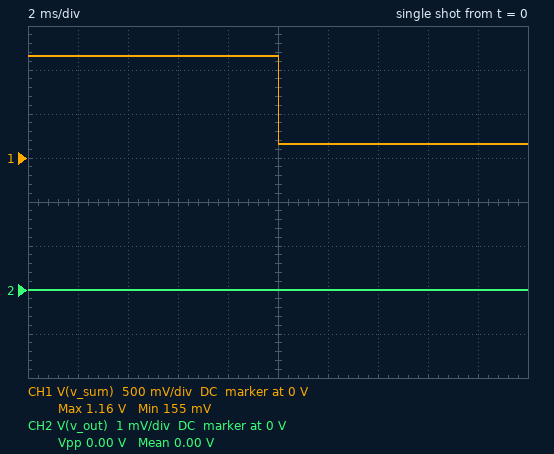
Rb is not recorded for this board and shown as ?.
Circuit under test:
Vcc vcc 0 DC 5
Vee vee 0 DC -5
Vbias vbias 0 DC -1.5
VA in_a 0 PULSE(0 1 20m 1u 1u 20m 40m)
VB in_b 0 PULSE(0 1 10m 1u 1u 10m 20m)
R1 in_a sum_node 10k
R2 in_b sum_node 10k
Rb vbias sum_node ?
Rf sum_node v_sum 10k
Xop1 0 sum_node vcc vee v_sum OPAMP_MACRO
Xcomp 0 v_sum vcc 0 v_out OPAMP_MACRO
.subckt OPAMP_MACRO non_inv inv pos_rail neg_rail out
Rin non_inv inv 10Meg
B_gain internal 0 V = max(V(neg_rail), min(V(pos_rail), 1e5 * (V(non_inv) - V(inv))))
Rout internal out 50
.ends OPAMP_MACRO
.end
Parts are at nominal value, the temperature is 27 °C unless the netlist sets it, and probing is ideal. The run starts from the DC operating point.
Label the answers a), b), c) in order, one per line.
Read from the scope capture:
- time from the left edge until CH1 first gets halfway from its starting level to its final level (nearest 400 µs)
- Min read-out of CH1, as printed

a) 10.0 ms
b) 155 mV
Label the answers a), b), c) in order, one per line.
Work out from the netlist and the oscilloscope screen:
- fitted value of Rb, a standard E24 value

a) 13 kΩ
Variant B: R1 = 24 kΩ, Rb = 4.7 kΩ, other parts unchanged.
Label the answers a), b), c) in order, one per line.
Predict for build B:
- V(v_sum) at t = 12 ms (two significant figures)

a) 2.2 V
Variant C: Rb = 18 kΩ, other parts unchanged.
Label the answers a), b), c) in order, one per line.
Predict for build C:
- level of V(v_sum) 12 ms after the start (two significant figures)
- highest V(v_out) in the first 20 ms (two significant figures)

a) -170 mV
b) 5.0 V
